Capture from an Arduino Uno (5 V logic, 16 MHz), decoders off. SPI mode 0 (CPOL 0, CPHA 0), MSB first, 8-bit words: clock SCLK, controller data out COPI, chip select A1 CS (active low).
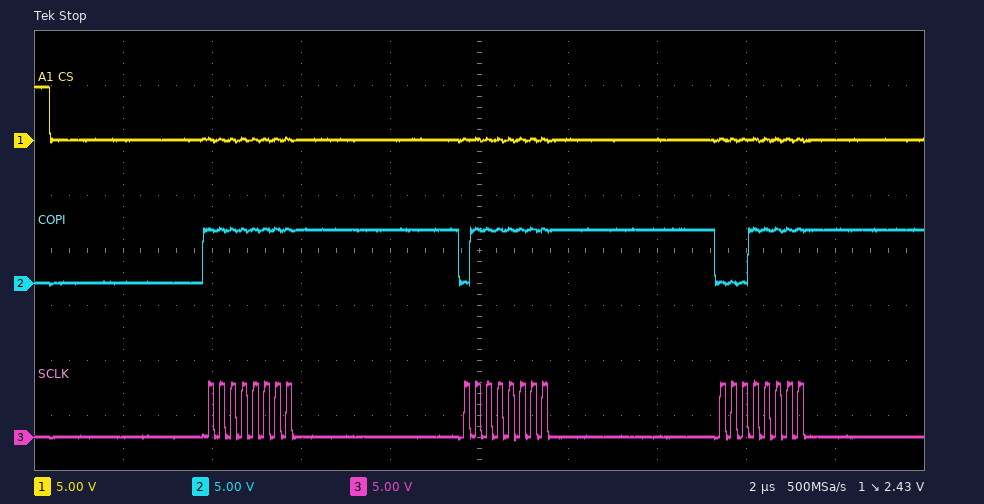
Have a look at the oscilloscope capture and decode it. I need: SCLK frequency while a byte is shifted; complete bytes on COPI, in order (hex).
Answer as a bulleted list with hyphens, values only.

- 4 MHz
- FF 7F 1F
